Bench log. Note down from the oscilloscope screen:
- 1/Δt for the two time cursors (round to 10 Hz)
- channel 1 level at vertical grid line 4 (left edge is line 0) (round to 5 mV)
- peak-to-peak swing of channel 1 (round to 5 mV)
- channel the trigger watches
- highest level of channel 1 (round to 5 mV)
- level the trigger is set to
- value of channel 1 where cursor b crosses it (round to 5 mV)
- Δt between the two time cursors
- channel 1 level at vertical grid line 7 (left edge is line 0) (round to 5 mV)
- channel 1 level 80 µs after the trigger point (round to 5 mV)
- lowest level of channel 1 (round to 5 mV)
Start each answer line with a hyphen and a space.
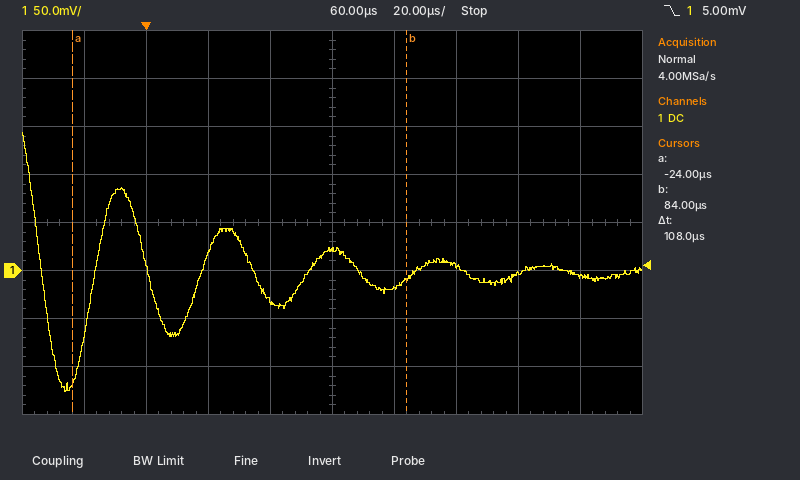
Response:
- 9.26 kHz
- -30 mV
- 270 mV
- channel 1
- 145 mV
- 5.00 mV
- -10 mV
- 108 µs
- 5 mV
- -20 mV
- -125 mV
